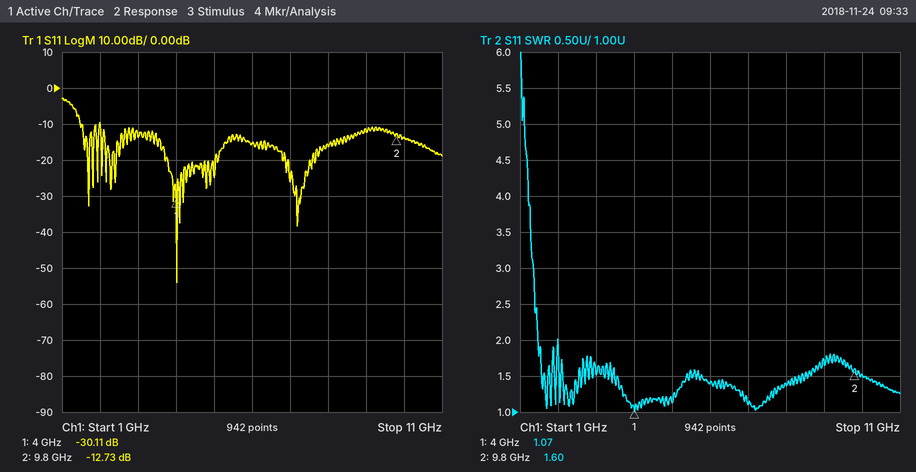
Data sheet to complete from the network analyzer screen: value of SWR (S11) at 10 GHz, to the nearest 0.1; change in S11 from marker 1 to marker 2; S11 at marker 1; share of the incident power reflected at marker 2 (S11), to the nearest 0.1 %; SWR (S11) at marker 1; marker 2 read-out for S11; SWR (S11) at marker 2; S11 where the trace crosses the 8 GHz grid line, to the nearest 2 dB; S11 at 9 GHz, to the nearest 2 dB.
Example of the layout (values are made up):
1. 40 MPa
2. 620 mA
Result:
1. 1.5
2. 17.38 dB
3. -30.11 dB
4. 5.3 %
5. 1.07
6. -12.73 dB
7. 1.60
8. -16 dB
9. -12 dB
